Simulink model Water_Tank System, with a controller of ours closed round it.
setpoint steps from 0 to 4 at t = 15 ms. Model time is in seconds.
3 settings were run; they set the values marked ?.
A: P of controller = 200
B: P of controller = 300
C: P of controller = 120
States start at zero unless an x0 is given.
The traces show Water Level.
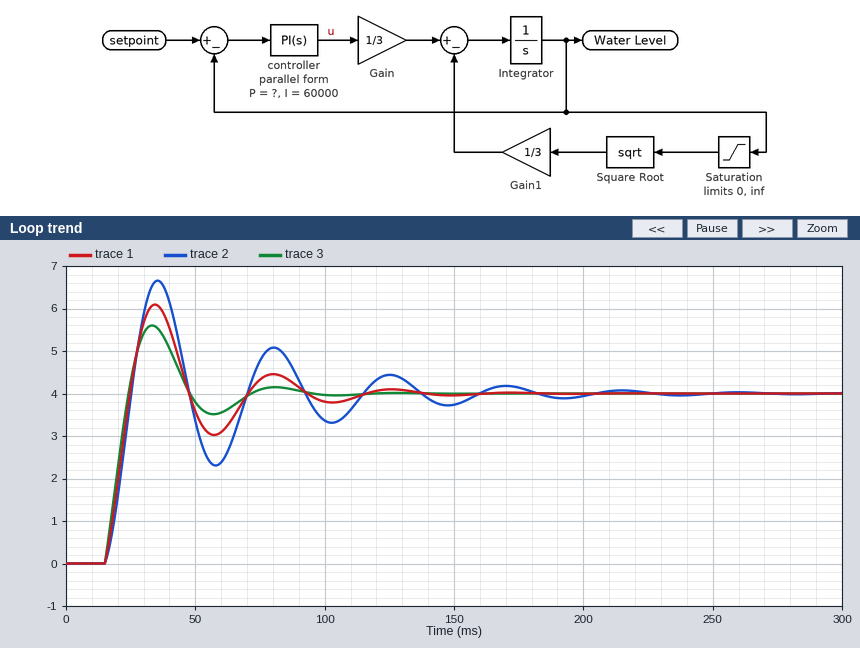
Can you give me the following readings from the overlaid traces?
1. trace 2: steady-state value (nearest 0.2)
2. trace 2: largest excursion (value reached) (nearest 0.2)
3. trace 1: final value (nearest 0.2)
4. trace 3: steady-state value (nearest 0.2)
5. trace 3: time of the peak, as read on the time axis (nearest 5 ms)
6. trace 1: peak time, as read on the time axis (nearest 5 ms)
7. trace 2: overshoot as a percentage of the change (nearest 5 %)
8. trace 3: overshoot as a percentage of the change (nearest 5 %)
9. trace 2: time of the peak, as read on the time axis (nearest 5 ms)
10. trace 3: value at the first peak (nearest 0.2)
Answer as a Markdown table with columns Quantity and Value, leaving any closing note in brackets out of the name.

| Quantity | Value |
|---|---|
| trace 2: steady-state value | 4.0 |
| trace 2: largest excursion (value reached) | 6.6 |
| trace 1: final value | 4.0 |
| trace 3: steady-state value | 4.0 |
| trace 3: time of the peak, as read on the time axis | 35 ms |
| trace 1: peak time, as read on the time axis | 35 ms |
| trace 2: overshoot as a percentage of the change | 65 % |
| trace 3: overshoot as a percentage of the change | 40 % |
| trace 2: time of the peak, as read on the time axis | 35 ms |
| trace 3: value at the first peak | 5.6 |
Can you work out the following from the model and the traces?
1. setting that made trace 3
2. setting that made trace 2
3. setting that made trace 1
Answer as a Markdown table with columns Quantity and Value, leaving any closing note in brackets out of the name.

| Quantity | Value |
|---|---|
| setting that made trace 3 | B |
| setting that made trace 2 | C |
| setting that made trace 1 | A |
